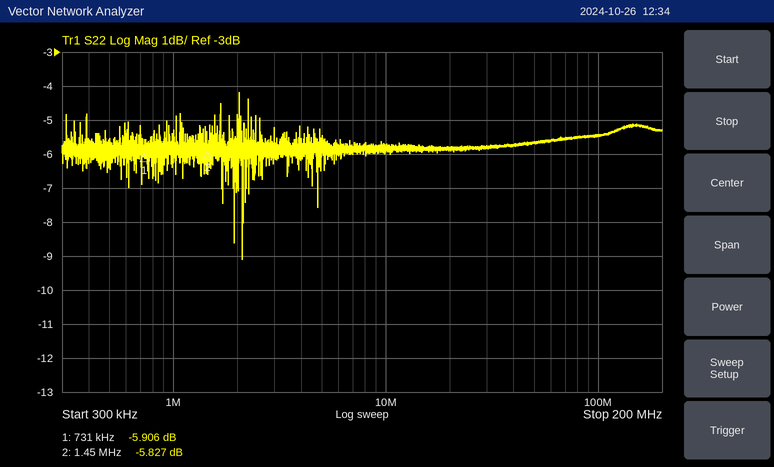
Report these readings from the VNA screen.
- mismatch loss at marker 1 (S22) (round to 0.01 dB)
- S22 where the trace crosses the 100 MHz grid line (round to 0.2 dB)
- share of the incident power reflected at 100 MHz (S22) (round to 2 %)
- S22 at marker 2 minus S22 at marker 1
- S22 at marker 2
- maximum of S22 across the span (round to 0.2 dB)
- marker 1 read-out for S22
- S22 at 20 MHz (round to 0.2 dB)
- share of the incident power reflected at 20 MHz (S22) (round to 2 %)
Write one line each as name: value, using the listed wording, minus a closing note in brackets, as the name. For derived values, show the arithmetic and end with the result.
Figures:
mismatch loss at marker 1 (S22): −10 log10(1 − 10^(-5.906/10)) ≈ 1.29 dB
S22 where the trace crosses the 100 MHz grid line: -5.4 dB
share of the incident power reflected at 100 MHz (S22): 10^(-5.4/10) ≈ 28.8 %, so 28 % to the nearest 2 %
S22 at marker 2 minus S22 at marker 1: -5.827 − (-5.906) = 0.079 dB
S22 at marker 2: -5.827 dB
maximum of S22 across the span: -4.2 dB
marker 1 read-out for S22: -5.906 dB
S22 at 20 MHz: -5.8 dB
share of the incident power reflected at 20 MHz (S22): 10^(-5.8/10) ≈ 26 %
